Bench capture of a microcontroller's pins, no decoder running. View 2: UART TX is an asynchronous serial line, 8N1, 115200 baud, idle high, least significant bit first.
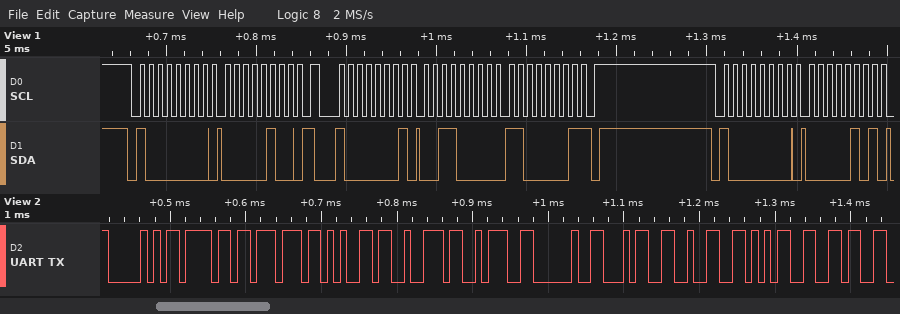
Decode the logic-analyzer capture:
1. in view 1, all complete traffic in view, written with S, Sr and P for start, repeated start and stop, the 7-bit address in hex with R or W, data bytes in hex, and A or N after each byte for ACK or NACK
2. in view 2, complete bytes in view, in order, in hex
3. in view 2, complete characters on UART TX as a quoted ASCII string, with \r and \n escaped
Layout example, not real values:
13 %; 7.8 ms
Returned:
S 40W A 04 A Sr 40R A 30 A C1 N P S 40W A 05 A; 50 6F 77 65 72 3A 20 34 32 35 36; "Power: 4256"
